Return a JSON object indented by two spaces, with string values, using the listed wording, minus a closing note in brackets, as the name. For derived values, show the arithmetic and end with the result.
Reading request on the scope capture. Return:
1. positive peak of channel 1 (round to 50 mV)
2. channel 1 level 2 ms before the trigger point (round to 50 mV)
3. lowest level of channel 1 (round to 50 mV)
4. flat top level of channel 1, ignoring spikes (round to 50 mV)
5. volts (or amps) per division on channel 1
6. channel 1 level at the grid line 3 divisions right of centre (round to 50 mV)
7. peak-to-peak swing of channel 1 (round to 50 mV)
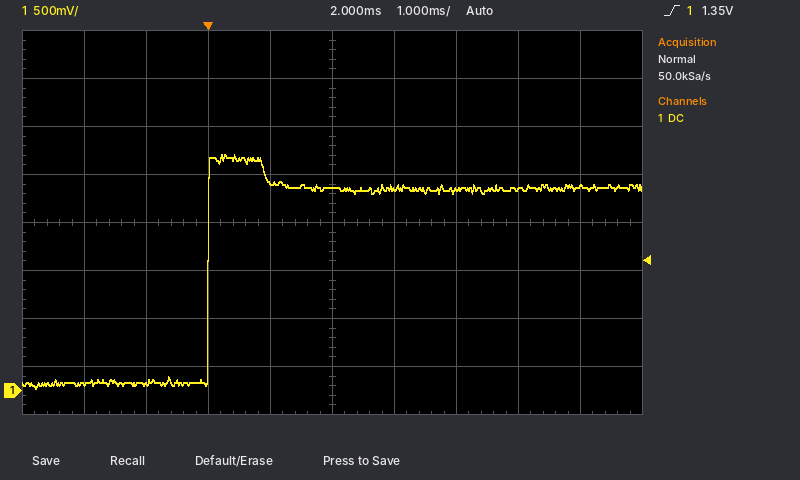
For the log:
{
  "positive peak of channel 1": "2.45 V",
  "channel 1 level 2 ms before the trigger point": "50 mV",
  "lowest level of channel 1": "0 mV",
  "flat top level of channel 1, ignoring spikes": "2.10 V",
  "volts (or amps) per division on channel 1": "500 mV",
  "channel 1 level at the grid line 3 divisions right of centre": "2.10 V",
  "peak-to-peak swing of channel 1": "2.45 V − (0 mV) = 2.45 V"
}
